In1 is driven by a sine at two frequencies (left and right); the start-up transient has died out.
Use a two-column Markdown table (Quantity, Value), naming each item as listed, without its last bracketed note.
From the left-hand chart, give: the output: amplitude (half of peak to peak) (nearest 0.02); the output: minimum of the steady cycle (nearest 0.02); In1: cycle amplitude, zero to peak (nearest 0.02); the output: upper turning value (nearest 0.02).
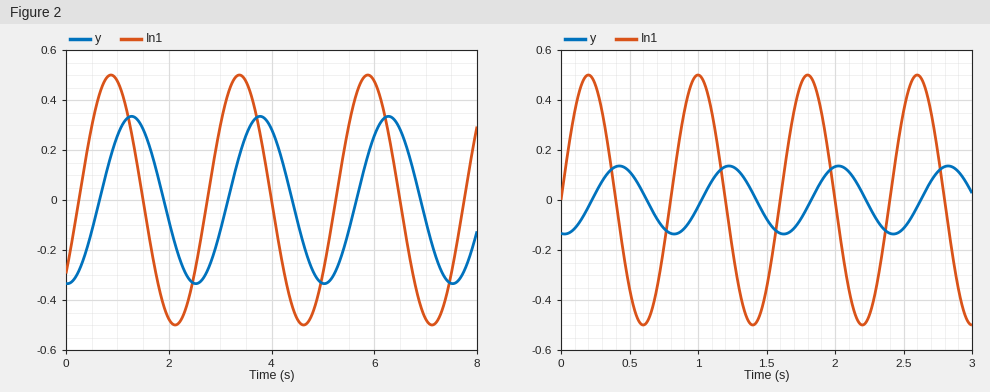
| Quantity | Value |
|---|---|
| the output: amplitude (half of peak to peak) | 0.34 |
| the output: minimum of the steady cycle | -0.34 |
| In1: cycle amplitude, zero to peak | 0.50 |
| the output: upper turning value | 0.34 |
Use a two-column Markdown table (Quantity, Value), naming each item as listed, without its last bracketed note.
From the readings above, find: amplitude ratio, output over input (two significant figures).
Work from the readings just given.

| Quantity | Value |
|---|---|
| amplitude ratio, output over input | 0.68 |
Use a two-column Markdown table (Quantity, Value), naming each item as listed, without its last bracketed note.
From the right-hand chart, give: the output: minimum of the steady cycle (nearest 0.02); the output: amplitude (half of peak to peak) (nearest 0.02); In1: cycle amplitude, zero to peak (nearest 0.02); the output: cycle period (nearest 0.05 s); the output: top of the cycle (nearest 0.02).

| Quantity | Value |
|---|---|
| the output: minimum of the steady cycle | -0.14 |
| the output: amplitude (half of peak to peak) | 0.14 |
| In1: cycle amplitude, zero to peak | 0.50 |
| the output: cycle period | 0.80 s |
| the output: top of the cycle | 0.14 |
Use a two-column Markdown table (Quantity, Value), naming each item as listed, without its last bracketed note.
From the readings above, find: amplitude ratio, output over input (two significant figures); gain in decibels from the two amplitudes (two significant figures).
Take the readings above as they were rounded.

| Quantity | Value |
|---|---|
| amplitude ratio, output over input | 0.28 |
| gain in decibels from the two amplitudes | -11 dB |
